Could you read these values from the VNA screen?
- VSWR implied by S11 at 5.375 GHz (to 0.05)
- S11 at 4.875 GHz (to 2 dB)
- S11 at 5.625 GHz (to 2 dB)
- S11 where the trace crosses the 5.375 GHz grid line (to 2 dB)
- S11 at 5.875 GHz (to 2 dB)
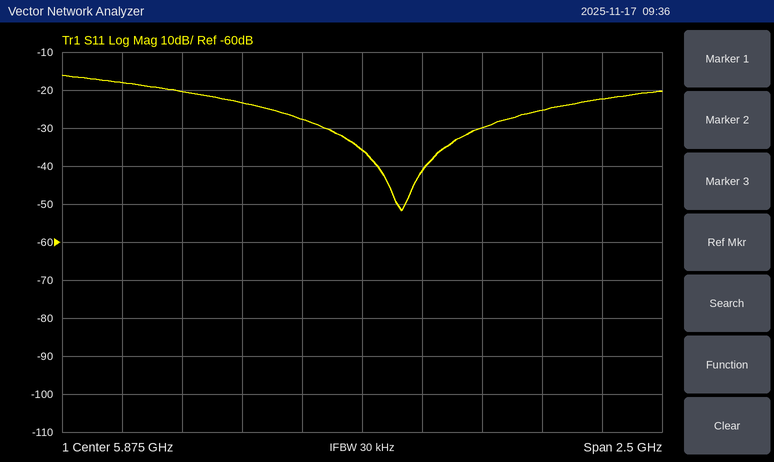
1.15
-18 dB
-28 dB
-24 dB
-36 dB
